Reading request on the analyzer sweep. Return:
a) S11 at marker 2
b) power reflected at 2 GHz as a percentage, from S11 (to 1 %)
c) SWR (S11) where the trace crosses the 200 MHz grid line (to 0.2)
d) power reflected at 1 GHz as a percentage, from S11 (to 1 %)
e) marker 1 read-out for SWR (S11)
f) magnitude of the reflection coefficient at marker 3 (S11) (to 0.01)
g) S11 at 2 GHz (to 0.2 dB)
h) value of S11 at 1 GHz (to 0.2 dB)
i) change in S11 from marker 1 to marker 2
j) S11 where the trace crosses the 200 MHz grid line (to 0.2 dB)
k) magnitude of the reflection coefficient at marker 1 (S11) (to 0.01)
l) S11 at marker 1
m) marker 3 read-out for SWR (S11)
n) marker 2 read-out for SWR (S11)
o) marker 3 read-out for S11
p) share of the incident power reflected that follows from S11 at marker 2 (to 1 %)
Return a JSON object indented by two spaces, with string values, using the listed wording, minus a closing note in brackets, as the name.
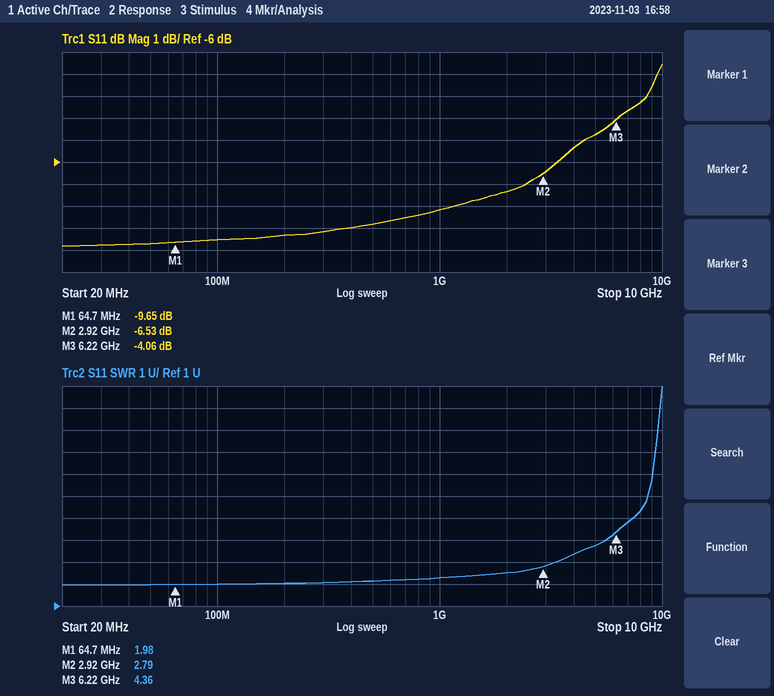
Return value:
{
  "S11 at marker 2": "-6.53 dB",
  "power reflected at 2 GHz as a percentage, from S11": "18 %",
  "SWR (S11) where the trace crosses the 200 MHz grid line": "2.0",
  "power reflected at 1 GHz as a percentage, from S11": "15 %",
  "marker 1 read-out for SWR": "1.98",
  "magnitude of the reflection coefficient at marker 3 (S11)": "0.63",
  "S11 at 2 GHz": "-7.4 dB",
  "value of S11 at 1 GHz": "-8.2 dB",
  "change in S11 from marker 1 to marker 2": "3.12 dB",
  "S11 where the trace crosses the 200 MHz grid line": "-9.4 dB",
  "magnitude of the reflection coefficient at marker 1 (S11)": "0.33",
  "S11 at marker 1": "-9.65 dB",
  "marker 3 read-out for SWR": "4.36",
  "marker 2 read-out for SWR": "2.79",
  "marker 3 read-out for S11": "-4.06 dB",
  "share of the incident power reflected that follows from S11 at marker 2": "22 %"
}
